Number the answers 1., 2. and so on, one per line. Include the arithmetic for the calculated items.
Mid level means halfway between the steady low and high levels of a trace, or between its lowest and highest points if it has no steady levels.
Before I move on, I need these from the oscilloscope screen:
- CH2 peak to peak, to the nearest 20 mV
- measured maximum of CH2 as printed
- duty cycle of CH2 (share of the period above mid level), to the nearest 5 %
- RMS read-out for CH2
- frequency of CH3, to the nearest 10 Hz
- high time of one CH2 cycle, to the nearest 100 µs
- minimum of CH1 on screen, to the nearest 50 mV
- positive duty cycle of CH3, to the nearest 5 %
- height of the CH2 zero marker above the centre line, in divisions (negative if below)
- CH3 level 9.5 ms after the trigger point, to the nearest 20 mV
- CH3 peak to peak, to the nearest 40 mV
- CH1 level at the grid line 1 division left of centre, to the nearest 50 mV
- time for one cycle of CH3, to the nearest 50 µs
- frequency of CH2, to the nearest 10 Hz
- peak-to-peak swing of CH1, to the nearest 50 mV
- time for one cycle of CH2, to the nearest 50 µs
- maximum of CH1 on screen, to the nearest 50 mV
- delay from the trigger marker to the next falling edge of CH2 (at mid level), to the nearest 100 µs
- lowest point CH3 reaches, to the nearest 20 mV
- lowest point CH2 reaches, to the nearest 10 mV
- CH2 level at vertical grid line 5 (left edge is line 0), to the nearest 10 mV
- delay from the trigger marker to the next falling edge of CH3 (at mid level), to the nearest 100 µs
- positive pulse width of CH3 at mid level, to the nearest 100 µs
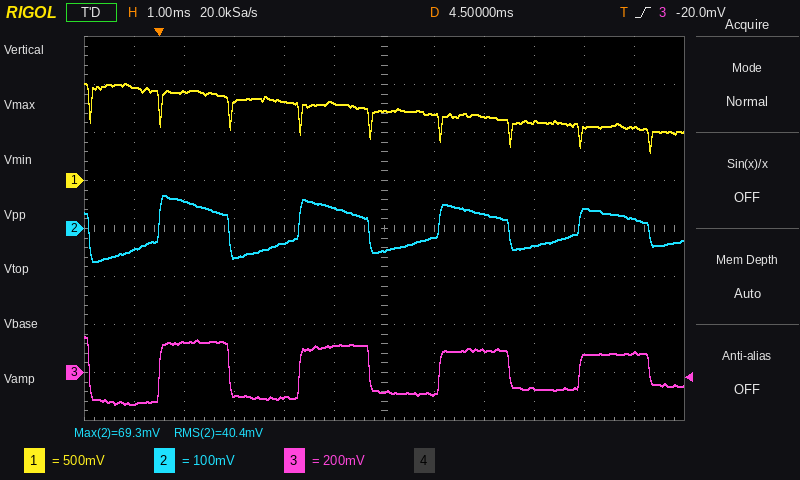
1. 140 mV
2. 69.3 mV
3. 1.4 ms / 2.80 ms ≈ 50 %
4. 40.4 mV
5. 1 / 2.80 ms ≈ 357 Hz, so 360 Hz to the nearest 10 Hz
6. 1.4 ms
7. 300 mV
8. 1.4 ms / 2.80 ms ≈ 50 %
9. 0.0 div
10. 80 mV
11. 280 mV
12. 800 mV
13. 2.80 ms
14. 1 / 2.80 ms ≈ 357 Hz, so 360 Hz to the nearest 10 Hz
15. 1.00 V − (300 mV) = 700 mV
16. 2.80 ms
17. 1.00 V
18. 1.4 ms
19. -140 mV
20. -70 mV
21. 40 mV
22. 1.4 ms
23. 1.4 ms
